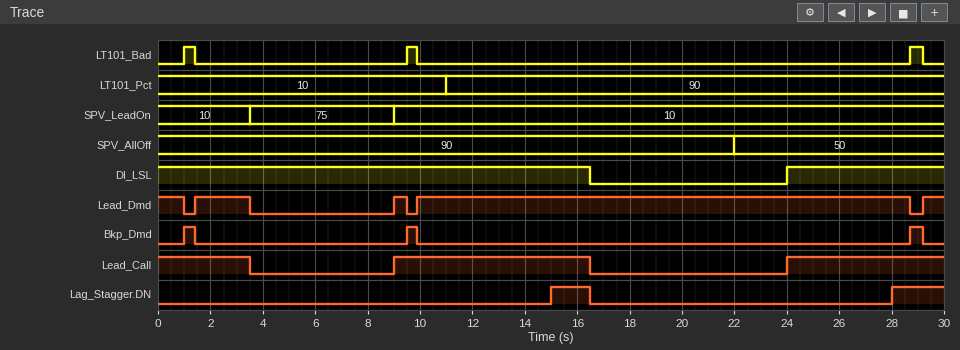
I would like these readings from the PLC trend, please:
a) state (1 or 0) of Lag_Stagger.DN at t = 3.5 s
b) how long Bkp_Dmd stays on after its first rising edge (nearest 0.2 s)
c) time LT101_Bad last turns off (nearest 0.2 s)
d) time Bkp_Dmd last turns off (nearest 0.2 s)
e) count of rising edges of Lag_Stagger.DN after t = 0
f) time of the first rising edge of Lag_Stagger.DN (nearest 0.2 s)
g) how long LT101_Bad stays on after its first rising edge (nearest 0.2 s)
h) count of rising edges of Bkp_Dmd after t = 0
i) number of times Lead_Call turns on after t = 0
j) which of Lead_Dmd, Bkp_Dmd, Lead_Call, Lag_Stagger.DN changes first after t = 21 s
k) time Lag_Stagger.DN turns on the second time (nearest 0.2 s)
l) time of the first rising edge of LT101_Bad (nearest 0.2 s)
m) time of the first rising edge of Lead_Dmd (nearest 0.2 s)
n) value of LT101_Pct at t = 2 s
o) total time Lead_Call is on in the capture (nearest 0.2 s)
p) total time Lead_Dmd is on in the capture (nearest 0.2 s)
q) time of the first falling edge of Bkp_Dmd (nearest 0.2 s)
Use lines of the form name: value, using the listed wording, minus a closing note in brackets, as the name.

state (1 or 0) of Lag_Stagger.DN at t = 3.5 s: 0
how long Bkp_Dmd stays on after its first rising edge: 0.4 s
time LT101_Bad last turns off: 29.2 s
time Bkp_Dmd last turns off: 29.2 s
count of rising edges of Lag_Stagger.DN after t = 0: 2
time of the first rising edge of Lag_Stagger.DN: 15.0 s
how long LT101_Bad stays on after its first rising edge: 0.4 s
count of rising edges of Bkp_Dmd after t = 0: 3
number of times Lead_Call turns on after t = 0: 2
which of Lead_Dmd, Bkp_Dmd, Lead_Call, Lag_Stagger.DN changes first after t = 21 s: Lead_Call
time Lag_Stagger.DN turns on the second time: 28.0 s
time of the first rising edge of LT101_Bad: 1.0 s
time of the first rising edge of Lead_Dmd: 1.4 s
value of LT101_Pct at t = 2 s: 10
total time Lead_Call is on in the capture: 17.0 s
total time Lead_Dmd is on in the capture: 23.2 s
time of the first falling edge of Bkp_Dmd: 1.4 s
